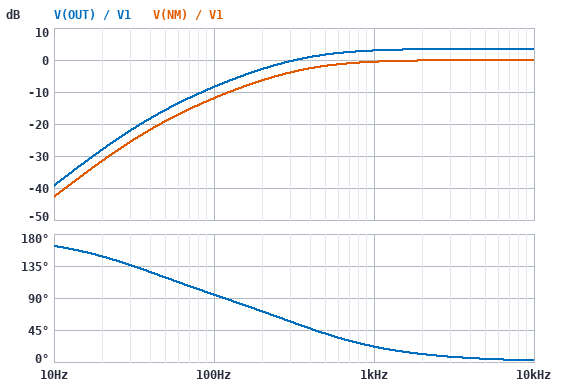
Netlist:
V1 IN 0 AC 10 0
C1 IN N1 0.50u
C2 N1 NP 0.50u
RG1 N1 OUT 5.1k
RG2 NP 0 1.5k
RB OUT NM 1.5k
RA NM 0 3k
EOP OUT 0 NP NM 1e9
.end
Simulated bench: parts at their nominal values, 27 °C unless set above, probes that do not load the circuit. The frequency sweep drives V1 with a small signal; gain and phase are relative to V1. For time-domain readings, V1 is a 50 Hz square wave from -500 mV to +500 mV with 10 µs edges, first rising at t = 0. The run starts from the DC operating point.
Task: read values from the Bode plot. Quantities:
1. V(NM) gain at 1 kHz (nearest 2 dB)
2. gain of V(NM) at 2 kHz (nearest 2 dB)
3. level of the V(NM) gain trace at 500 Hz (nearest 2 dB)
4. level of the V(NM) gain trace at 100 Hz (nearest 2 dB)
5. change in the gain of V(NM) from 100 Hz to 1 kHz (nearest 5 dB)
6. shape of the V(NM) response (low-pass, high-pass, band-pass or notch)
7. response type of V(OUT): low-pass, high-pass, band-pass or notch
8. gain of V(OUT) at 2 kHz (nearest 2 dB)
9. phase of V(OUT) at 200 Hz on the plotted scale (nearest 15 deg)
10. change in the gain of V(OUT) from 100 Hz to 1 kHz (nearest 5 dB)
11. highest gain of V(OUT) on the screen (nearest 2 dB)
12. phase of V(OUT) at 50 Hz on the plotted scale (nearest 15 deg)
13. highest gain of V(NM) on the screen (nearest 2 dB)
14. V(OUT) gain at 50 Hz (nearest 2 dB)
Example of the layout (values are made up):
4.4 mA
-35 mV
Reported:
0 dB
0 dB
-2 dB
-12 dB
10 dB
high-pass
high-pass
4 dB
75 deg
10 dB
4 dB
120 deg
0 dB
-16 dB
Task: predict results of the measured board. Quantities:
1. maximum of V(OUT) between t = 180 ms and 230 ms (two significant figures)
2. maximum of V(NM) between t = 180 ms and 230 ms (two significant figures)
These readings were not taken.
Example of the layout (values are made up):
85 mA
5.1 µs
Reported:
1.5 V
1.0 V
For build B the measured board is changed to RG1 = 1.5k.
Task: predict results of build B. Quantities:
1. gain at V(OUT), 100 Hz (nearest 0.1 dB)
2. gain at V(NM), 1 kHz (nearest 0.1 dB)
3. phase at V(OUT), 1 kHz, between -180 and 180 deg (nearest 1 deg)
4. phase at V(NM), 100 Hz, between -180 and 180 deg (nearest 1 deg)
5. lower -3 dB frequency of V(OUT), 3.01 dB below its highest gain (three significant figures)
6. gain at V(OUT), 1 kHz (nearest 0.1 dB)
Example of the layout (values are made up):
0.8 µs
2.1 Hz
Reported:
-10.0 dB
-0.1 dB
18 deg
138 deg
226 Hz
3.5 dB
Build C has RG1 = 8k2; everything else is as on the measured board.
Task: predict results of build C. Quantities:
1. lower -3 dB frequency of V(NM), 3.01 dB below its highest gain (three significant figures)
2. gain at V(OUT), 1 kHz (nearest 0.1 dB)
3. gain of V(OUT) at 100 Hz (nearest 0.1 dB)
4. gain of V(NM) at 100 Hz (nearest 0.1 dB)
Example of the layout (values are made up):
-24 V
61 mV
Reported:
385 Hz
2.9 dB
-8.6 dB
-12.2 dB
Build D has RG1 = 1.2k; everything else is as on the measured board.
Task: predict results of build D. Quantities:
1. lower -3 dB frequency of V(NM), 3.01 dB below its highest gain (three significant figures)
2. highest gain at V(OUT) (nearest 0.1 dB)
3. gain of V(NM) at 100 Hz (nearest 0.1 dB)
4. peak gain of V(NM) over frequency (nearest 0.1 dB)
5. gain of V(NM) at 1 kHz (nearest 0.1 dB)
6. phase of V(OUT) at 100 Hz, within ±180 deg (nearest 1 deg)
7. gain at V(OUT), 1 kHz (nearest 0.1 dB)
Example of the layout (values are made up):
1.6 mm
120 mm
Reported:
215 Hz
3.8 dB
-14.8 dB
0.3 dB
0.1 dB
148 deg
3.6 dB
